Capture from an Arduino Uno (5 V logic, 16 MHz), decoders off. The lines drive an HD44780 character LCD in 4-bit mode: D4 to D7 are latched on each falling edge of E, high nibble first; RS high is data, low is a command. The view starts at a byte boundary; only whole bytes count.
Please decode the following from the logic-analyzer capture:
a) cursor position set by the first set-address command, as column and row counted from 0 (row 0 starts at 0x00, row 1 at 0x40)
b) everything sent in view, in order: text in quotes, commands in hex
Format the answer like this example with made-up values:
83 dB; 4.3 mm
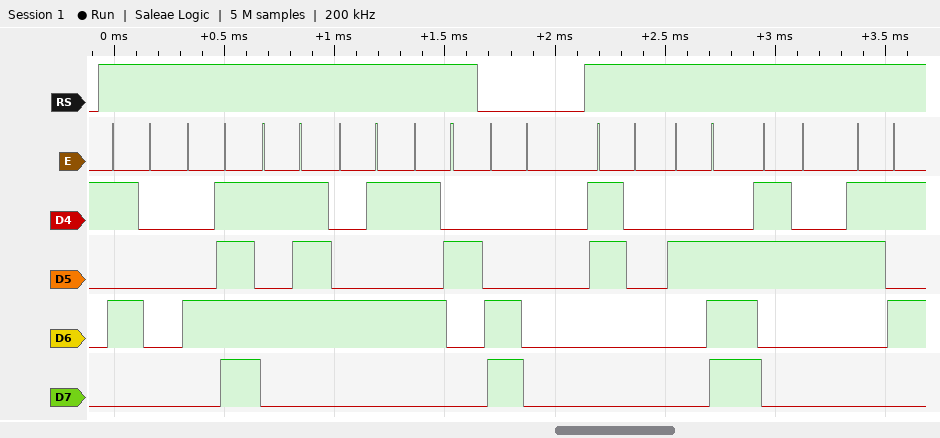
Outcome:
column 0, row 1; "POWER" 0xC0 "0.25"
